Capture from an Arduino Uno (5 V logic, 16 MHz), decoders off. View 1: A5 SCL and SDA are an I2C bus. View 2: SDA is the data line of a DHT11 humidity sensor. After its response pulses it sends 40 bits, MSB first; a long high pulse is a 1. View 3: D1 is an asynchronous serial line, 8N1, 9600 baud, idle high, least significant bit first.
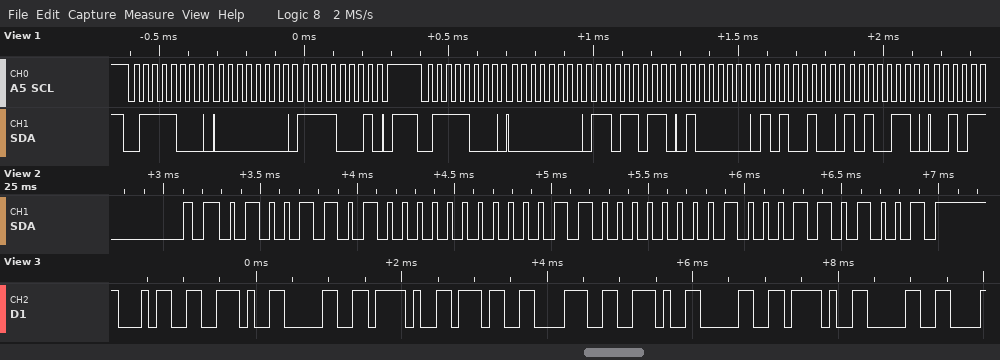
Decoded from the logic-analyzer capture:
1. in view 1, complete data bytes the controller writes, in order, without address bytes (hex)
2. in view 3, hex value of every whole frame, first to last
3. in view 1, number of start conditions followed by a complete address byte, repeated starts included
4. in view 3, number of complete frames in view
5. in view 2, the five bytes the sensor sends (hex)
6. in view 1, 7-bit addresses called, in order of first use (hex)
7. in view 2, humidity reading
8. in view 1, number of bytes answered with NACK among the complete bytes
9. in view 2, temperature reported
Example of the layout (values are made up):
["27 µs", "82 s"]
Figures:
["00 F1 00 DB 40 A4 A6", "34 2E 30 2F 37 38 2E 30 2F 30", "2", "10", "4D 00 18 04 69", "0x3C", "77 %", "0", "24.4 °C"]
